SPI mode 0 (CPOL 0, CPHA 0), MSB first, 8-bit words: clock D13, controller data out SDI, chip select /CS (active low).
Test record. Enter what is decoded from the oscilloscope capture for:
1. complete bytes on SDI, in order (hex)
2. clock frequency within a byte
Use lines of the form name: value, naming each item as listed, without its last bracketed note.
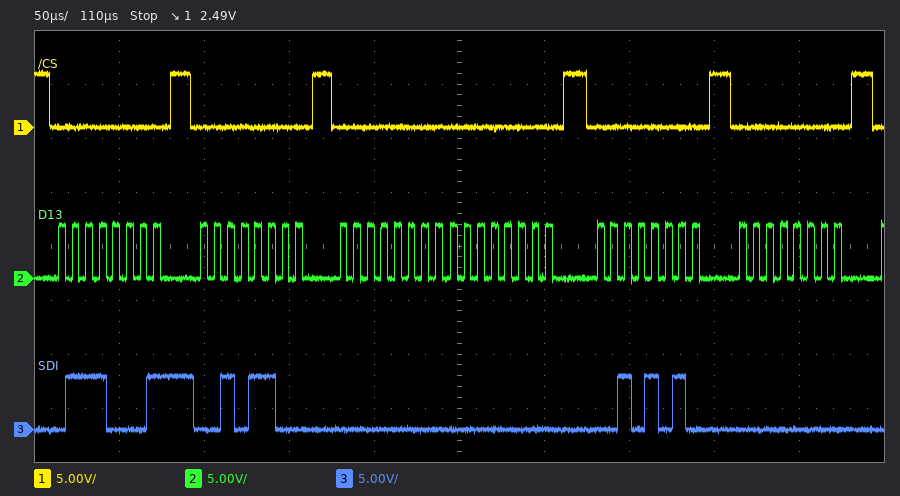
complete bytes on SDI, in order: 71 2C 00 00 2A 00
clock frequency within a byte: 125 kHz
